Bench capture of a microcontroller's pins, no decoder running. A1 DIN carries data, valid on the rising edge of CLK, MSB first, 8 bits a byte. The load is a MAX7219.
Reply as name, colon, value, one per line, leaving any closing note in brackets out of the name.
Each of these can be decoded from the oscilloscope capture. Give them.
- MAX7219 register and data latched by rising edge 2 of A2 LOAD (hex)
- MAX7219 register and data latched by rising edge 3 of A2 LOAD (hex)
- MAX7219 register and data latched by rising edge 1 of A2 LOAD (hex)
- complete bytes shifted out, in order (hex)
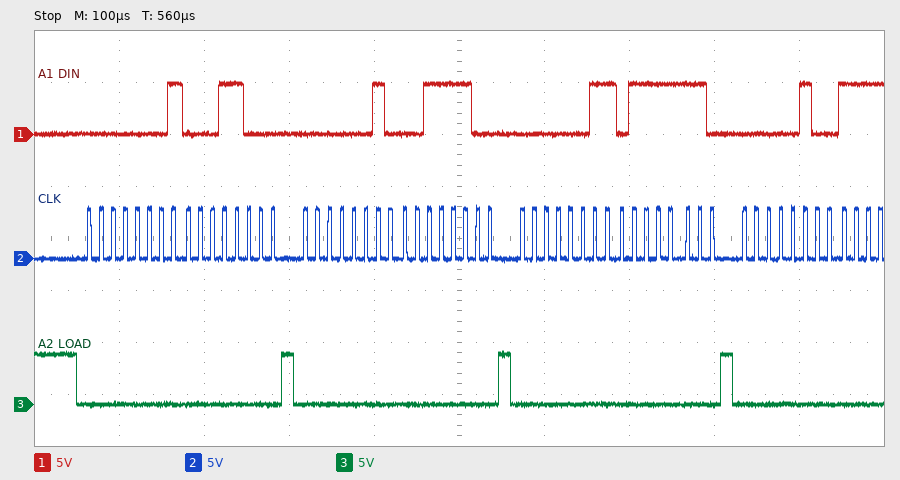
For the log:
MAX7219 register and data latched by rising edge 2 of A2 LOAD: register 0x2, data 0x3C
MAX7219 register and data latched by rising edge 3 of A2 LOAD: register 0x3, data 0x7E
MAX7219 register and data latched by rising edge 1 of A2 LOAD: register 0x1, data 0x18
complete bytes shifted out, in order: 01 18 02 3C 03 7E 04
